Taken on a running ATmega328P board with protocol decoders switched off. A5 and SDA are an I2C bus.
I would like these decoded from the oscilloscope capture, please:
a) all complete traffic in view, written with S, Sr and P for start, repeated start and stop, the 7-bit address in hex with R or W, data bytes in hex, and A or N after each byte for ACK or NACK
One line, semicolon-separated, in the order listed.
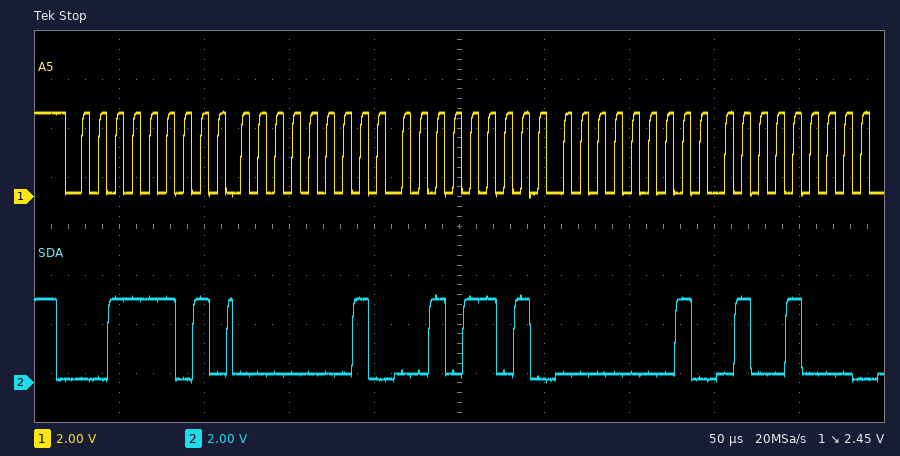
S 1ER A 01 A 2D A 01 A 48 A
